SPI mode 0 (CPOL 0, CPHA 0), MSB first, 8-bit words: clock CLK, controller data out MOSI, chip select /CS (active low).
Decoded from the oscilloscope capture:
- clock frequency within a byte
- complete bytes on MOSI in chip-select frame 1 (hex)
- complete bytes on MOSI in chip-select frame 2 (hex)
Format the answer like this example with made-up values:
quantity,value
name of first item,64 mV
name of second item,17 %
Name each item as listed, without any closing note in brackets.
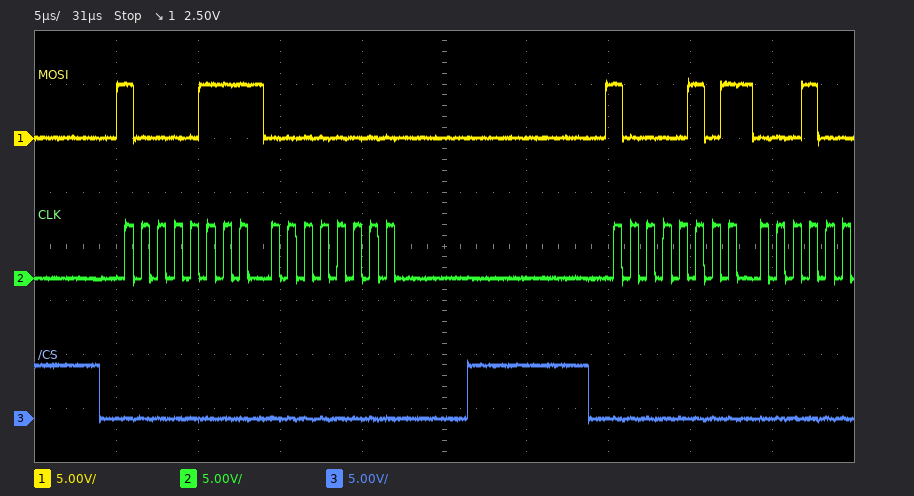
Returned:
quantity,value
clock frequency within a byte,1 MHz
complete bytes on MOSI in chip-select frame 1,87 00
complete bytes on MOSI in chip-select frame 2,85
